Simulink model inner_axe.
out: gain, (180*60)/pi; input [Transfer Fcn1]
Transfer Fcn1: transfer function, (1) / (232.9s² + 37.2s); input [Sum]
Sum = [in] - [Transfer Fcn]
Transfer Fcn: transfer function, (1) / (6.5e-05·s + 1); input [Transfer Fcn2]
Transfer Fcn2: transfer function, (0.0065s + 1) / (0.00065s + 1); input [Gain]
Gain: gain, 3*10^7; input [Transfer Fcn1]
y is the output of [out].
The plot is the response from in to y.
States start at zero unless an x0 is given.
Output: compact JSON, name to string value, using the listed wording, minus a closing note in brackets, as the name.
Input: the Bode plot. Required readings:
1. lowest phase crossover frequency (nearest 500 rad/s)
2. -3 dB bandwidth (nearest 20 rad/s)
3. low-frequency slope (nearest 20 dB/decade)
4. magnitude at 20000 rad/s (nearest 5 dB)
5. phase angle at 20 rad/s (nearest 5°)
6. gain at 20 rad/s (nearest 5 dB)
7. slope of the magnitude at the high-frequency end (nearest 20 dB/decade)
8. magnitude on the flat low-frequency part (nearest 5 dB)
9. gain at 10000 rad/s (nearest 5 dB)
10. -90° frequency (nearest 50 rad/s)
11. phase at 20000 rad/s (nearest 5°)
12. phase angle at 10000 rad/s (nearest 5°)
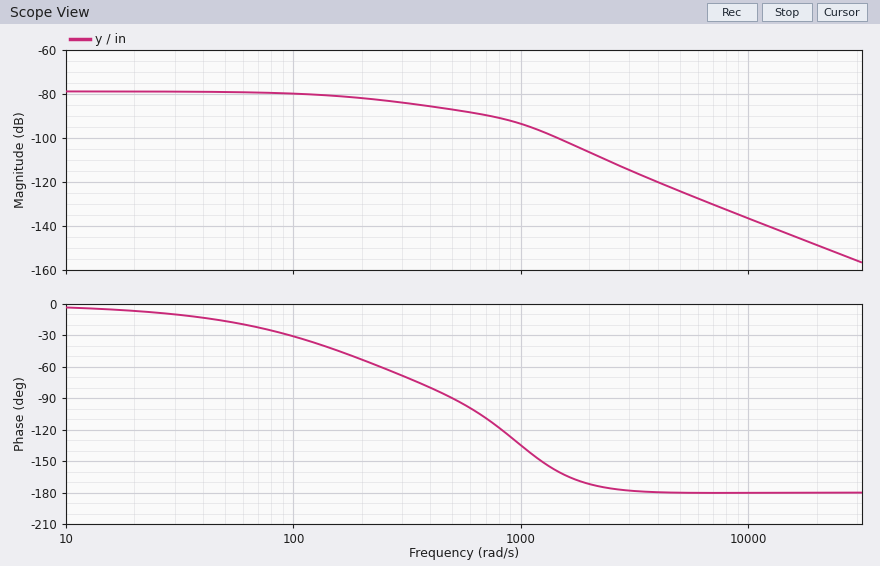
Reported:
{"lowest phase crossover frequency": "4500 rad/s", "-3 dB bandwidth": "200 rad/s", "low-frequency slope": "0 dB/decade", "magnitude at 20000 rad/s": "-150 dB", "phase angle at 20 rad/s": "-5°", "gain at 20 rad/s": "-80 dB", "slope of the magnitude at the high-frequency end": "-40 dB/decade", "magnitude on the flat low-frequency part": "-80 dB", "gain at 10000 rad/s": "-135 dB", "-90° frequency": "500 rad/s", "phase at 20000 rad/s": "-180°", "phase angle at 10000 rad/s": "-180°"}
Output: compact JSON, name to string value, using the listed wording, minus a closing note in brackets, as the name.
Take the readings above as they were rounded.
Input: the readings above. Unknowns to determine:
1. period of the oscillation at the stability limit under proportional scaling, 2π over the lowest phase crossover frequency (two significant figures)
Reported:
{"period of the oscillation at the stability limit under proportional scaling, 2π over the lowest phase crossover frequency": "0.0014 s"}
